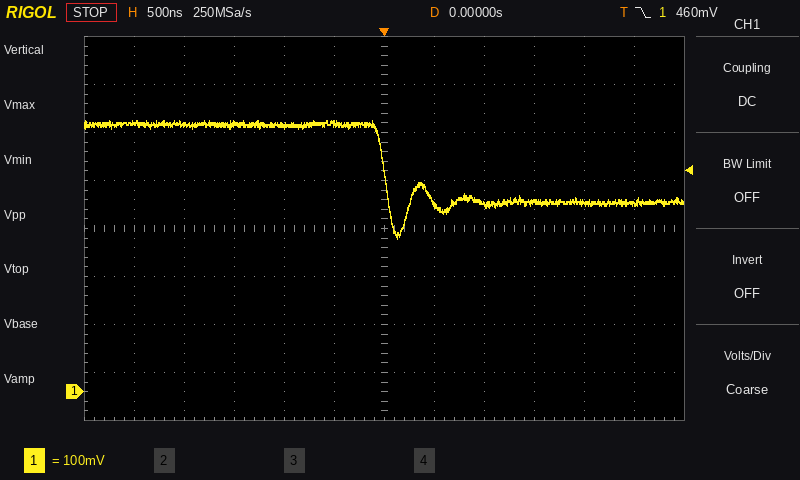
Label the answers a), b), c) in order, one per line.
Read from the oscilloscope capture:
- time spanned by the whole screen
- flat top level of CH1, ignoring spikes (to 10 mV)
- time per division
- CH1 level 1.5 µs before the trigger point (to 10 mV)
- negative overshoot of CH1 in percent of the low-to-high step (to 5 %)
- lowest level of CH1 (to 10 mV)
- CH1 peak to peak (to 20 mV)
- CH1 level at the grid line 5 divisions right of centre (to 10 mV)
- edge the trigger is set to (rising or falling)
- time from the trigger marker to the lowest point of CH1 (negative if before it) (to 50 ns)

a) 6 µs
b) 560 mV
c) 500 ns
d) 560 mV
e) 45 %
f) 320 mV
g) 240 mV
h) 390 mV
i) falling
j) +150 ns
